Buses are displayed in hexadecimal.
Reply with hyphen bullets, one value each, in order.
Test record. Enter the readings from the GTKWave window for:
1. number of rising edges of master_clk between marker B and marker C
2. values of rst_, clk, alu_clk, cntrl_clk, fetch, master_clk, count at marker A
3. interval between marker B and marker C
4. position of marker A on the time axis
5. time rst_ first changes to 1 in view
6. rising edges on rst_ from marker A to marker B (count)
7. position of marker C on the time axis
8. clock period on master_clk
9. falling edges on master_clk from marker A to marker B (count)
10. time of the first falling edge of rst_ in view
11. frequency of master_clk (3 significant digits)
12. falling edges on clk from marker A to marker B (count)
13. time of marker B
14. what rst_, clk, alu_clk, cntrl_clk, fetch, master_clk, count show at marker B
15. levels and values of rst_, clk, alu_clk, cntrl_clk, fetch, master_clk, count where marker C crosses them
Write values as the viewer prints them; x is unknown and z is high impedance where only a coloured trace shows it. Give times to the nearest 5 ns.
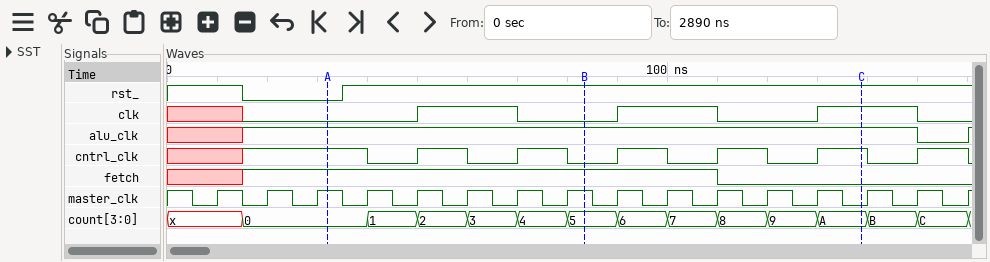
- 5
- rst_=0, clk=0, alu_clk=1, cntrl_clk=1, fetch=1, master_clk=1, count=0
- 55 ns
- 30 ns
- 35 ns
- 1
- 140 ns
- 10 ns
- 5
- 15 ns
- 100 MHz
- 1
- 85 ns
- rst_=1, clk=0, alu_clk=1, cntrl_clk=0, fetch=1, master_clk=1, count=5
- rst_=1, clk=1, alu_clk=1, cntrl_clk=1, fetch=0, master_clk=0, count=A
